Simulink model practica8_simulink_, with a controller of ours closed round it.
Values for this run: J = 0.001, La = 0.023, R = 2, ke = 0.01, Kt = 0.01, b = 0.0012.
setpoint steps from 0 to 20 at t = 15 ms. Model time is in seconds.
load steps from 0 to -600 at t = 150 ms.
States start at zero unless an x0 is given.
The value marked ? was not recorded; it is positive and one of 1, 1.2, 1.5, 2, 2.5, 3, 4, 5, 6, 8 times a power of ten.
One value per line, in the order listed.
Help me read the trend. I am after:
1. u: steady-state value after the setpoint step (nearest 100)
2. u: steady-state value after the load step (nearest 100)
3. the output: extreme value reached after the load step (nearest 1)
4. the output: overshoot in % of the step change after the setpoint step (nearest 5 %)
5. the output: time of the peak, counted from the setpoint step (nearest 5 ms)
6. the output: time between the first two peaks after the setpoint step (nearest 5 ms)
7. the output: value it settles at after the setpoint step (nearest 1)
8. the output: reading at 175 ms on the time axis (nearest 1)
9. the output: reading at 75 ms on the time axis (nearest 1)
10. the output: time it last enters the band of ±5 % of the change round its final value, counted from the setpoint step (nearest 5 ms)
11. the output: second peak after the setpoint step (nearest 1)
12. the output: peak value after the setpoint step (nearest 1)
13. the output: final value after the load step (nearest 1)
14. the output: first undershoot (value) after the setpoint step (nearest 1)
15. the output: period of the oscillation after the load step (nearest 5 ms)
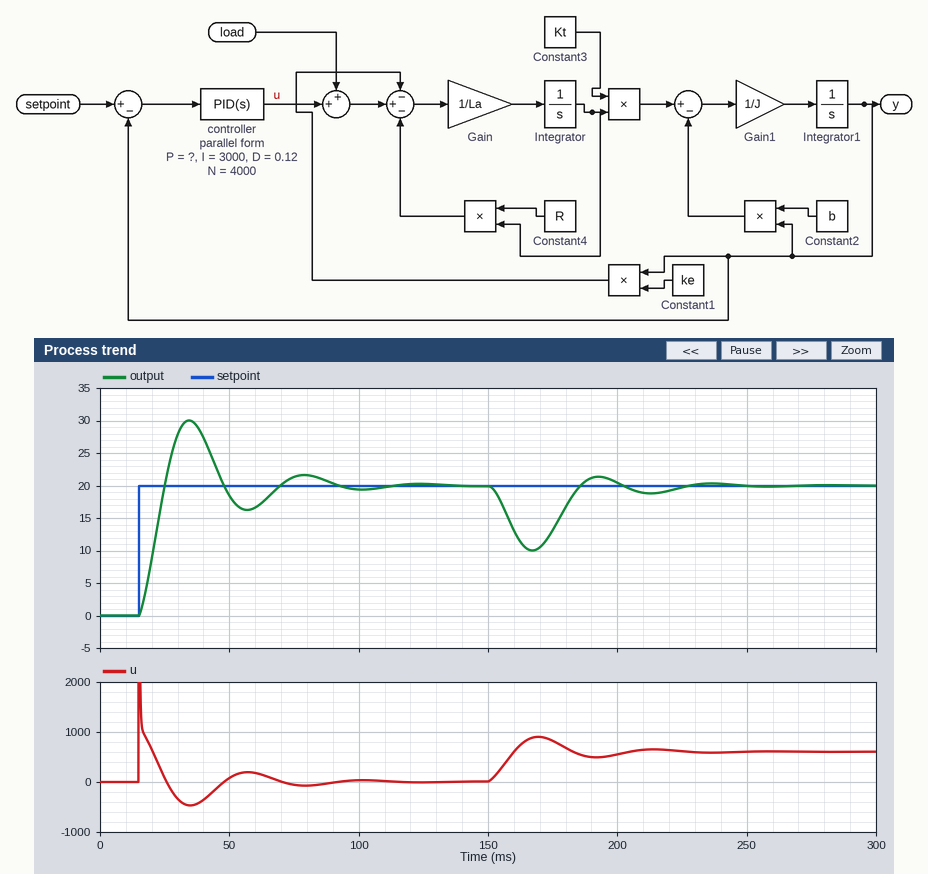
0
600
10
50 %
20 ms
45 ms
20
13
21
70 ms
22
30
20
16
45 ms
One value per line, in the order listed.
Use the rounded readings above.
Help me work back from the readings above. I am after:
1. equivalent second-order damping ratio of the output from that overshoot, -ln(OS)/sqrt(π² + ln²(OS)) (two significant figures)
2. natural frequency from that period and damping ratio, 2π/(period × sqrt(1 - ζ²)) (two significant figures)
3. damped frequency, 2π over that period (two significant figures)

0.22
0.14 rad/ms
0.14 rad/ms
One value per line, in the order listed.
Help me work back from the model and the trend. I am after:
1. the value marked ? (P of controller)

60
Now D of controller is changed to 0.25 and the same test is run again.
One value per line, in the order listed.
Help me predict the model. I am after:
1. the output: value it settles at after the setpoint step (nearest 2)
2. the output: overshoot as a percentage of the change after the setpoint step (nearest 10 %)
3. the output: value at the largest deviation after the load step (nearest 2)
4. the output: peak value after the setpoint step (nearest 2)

20
30 %
12
26
